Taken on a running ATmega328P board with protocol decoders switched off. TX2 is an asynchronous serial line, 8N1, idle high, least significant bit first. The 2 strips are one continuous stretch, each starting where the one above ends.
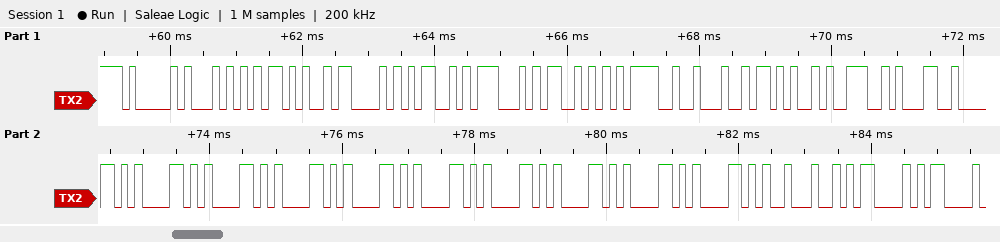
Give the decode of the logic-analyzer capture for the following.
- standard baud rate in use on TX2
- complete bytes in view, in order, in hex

9600 baud
0x41 0x54 0x2B 0x43 0x4D 0x47 0x53 0x3D 0x22 0x2B 0x39 0x31 0x58 0x58 0x58 0x58 0x58 0x58 0x58 0x58 0x58 0x58 0x22 0x0D 0x0D
